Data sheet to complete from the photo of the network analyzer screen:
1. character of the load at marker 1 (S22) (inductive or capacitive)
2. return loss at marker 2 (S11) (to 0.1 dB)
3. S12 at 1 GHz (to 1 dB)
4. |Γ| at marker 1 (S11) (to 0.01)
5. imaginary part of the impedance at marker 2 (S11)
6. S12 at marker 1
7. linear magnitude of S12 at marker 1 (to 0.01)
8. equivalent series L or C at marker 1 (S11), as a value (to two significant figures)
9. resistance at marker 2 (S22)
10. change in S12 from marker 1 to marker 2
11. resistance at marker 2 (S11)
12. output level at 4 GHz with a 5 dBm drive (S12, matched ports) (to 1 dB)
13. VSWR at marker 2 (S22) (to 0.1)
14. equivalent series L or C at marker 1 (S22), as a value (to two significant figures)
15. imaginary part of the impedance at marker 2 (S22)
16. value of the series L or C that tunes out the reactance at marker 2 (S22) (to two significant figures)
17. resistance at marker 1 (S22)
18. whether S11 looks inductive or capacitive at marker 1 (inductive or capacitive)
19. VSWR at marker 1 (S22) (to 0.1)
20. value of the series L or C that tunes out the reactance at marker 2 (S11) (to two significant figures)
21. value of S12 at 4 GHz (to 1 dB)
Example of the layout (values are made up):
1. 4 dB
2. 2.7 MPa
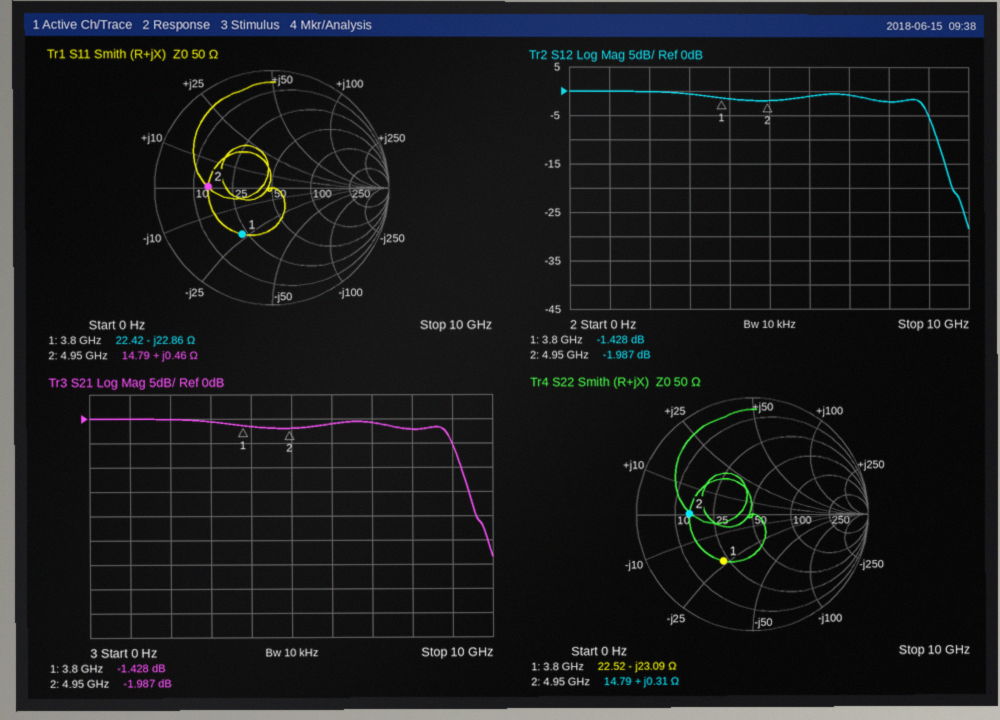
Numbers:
1. capacitive
2. 5.3 dB
3. 0 dB
4. 0.47
5. +0.46 Ω
6. -1.428 dB
7. 0.85
8. 1.8 pF
9. 14.79 Ω
10. -0.559 dB
11. 14.79 Ω
12. 3 dBm
13. 3.4
14. 1.8 pF
15. +0.31 Ω
16. 100 pF
17. 22.52 Ω
18. capacitive
19. 2.8
20. 70 pF
21. -2 dB
